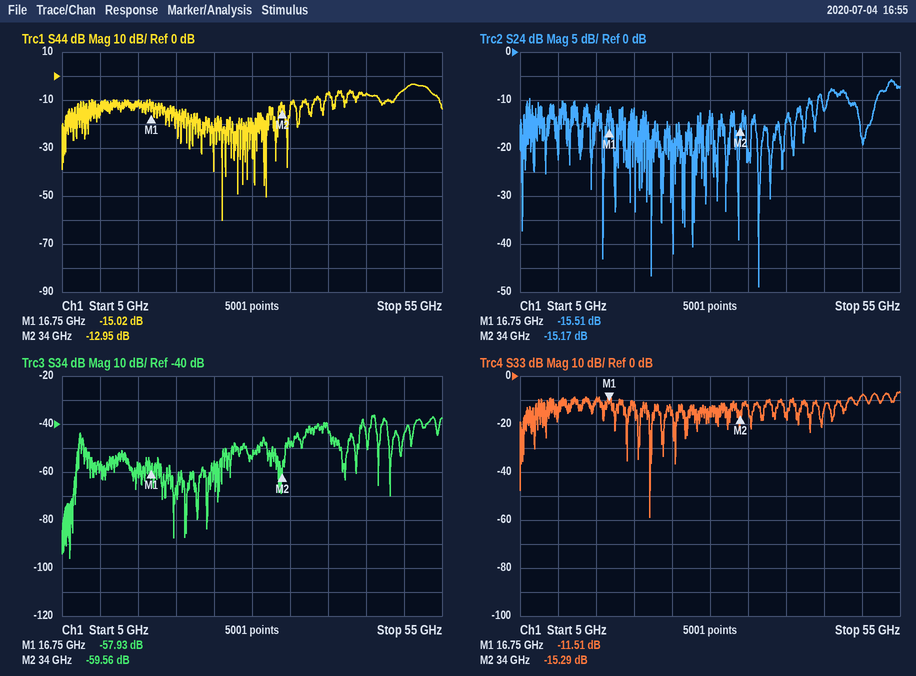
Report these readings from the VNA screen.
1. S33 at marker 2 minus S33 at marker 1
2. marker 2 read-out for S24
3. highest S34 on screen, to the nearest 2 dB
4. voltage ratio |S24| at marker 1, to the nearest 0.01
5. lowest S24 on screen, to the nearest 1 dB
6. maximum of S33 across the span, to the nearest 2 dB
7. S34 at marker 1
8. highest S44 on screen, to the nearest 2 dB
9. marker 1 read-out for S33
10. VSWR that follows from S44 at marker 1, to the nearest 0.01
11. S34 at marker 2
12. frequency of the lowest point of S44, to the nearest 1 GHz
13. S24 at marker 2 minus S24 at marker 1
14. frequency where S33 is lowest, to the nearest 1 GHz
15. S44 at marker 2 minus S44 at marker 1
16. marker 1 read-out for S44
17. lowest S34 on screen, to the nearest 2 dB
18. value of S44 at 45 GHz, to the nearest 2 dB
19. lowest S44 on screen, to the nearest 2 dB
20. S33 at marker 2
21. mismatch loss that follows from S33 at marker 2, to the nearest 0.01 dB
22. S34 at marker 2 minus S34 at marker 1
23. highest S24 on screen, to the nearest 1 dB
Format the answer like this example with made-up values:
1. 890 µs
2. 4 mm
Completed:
1. -3.78 dB
2. -15.17 dB
3. -36 dB
4. 0.17
5. -49 dB
6. -6 dB
7. -57.93 dB
8. -4 dB
9. -11.51 dB
10. 1.43
11. -59.56 dB
12. 26 GHz
13. 0.34 dB
14. 22 GHz
15. 2.07 dB
16. -15.02 dB
17. -96 dB
18. -8 dB
19. -60 dB
20. -15.29 dB
21. 0.13 dB
22. -1.63 dB
23. -6 dB
